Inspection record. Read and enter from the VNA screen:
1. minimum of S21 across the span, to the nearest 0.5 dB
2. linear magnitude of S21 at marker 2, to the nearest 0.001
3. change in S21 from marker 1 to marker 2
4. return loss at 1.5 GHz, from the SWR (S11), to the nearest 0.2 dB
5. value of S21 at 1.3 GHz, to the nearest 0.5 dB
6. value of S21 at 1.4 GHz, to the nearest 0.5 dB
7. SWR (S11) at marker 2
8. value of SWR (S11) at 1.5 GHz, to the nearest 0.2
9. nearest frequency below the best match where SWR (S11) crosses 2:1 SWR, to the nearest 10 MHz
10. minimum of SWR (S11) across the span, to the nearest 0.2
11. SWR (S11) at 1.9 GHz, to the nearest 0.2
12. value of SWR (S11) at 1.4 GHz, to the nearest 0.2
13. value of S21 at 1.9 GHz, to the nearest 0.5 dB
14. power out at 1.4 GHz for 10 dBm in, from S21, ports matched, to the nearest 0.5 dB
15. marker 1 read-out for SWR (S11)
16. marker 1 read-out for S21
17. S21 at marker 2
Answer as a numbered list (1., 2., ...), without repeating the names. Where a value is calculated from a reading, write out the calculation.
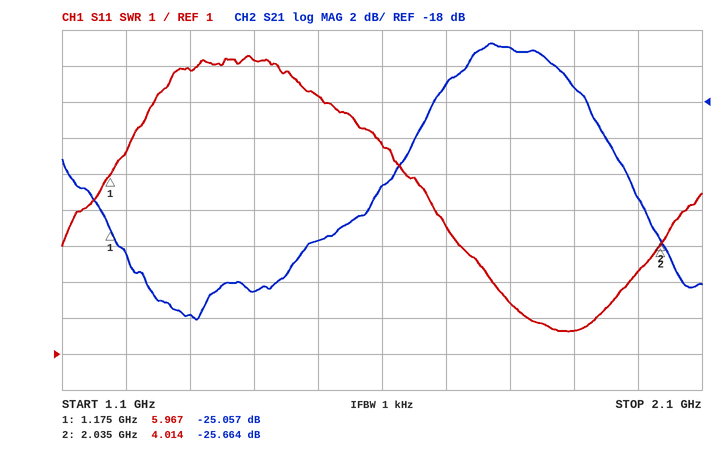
1. -30.0 dB
2. 10^(-25.664/20) ≈ 0.052
3. -25.664 − (-25.057) = -0.607 dB
4. −20 log10((8.2 − 1)/(8.2 + 1)) ≈ 2.13 dB, so 2.2 dB to the nearest 0.2 dB
5. -30.0 dB
6. -28.5 dB
7. 4.014
8. 8.2
9. 1.83 GHz
10. 1.6
11. 1.6
12. 9.2
13. -17.0 dB
14. 10 dBm + (-28.5 dB) = -18.5 dBm
15. 5.967
16. -25.057 dB
17. -25.664 dB
